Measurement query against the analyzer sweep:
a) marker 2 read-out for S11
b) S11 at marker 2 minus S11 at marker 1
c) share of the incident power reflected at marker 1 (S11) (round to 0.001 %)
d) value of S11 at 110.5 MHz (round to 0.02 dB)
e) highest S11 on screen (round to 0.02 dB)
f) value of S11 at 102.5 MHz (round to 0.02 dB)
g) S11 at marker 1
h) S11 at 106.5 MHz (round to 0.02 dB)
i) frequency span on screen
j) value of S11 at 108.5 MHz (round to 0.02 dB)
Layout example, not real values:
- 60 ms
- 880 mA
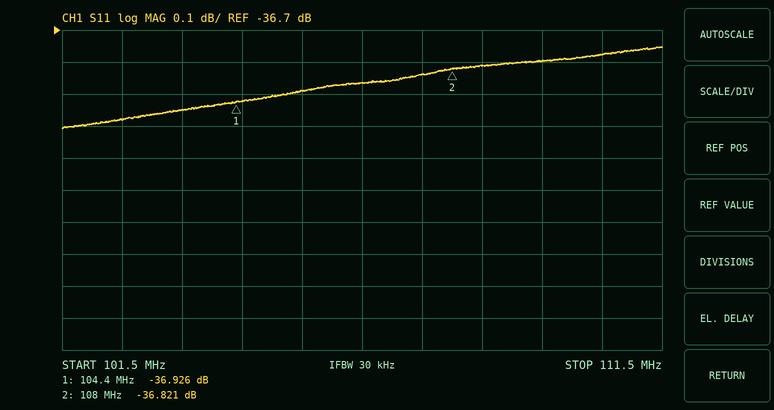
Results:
- -36.821 dB
- 0.105 dB
- 0.020 %
- -36.78 dB
- -36.76 dB
- -36.98 dB
- -36.926 dB
- -36.86 dB
- 10 MHz
- -36.82 dB
